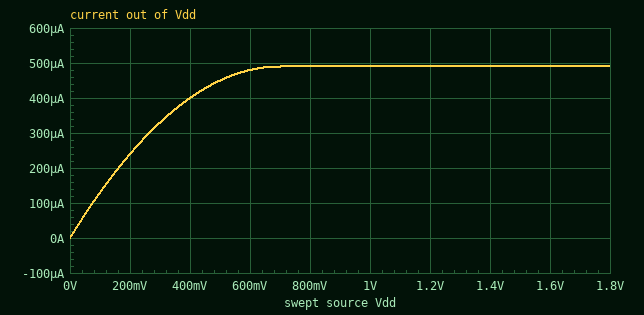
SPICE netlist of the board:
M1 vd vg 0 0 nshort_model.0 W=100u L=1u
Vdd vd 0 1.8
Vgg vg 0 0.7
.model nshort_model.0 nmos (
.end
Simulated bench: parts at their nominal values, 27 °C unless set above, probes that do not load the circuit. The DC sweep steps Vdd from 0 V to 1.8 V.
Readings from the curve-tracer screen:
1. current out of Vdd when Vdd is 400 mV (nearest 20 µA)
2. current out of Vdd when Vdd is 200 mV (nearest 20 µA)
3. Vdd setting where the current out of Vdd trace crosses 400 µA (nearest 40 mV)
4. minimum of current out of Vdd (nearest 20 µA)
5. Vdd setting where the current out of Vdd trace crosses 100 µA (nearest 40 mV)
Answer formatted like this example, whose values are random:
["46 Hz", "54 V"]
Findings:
["400 µA", "240 µA", "400 mV", "0 A", "80 mV"]
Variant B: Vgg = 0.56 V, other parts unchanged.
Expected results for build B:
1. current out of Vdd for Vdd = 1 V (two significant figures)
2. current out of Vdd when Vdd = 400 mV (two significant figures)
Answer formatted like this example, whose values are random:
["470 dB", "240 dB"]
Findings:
["310 µA", "290 µA"]
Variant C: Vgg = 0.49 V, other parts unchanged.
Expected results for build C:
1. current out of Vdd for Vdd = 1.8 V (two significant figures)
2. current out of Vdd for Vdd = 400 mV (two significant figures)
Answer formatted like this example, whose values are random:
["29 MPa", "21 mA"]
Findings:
["240 µA", "230 µA"]
